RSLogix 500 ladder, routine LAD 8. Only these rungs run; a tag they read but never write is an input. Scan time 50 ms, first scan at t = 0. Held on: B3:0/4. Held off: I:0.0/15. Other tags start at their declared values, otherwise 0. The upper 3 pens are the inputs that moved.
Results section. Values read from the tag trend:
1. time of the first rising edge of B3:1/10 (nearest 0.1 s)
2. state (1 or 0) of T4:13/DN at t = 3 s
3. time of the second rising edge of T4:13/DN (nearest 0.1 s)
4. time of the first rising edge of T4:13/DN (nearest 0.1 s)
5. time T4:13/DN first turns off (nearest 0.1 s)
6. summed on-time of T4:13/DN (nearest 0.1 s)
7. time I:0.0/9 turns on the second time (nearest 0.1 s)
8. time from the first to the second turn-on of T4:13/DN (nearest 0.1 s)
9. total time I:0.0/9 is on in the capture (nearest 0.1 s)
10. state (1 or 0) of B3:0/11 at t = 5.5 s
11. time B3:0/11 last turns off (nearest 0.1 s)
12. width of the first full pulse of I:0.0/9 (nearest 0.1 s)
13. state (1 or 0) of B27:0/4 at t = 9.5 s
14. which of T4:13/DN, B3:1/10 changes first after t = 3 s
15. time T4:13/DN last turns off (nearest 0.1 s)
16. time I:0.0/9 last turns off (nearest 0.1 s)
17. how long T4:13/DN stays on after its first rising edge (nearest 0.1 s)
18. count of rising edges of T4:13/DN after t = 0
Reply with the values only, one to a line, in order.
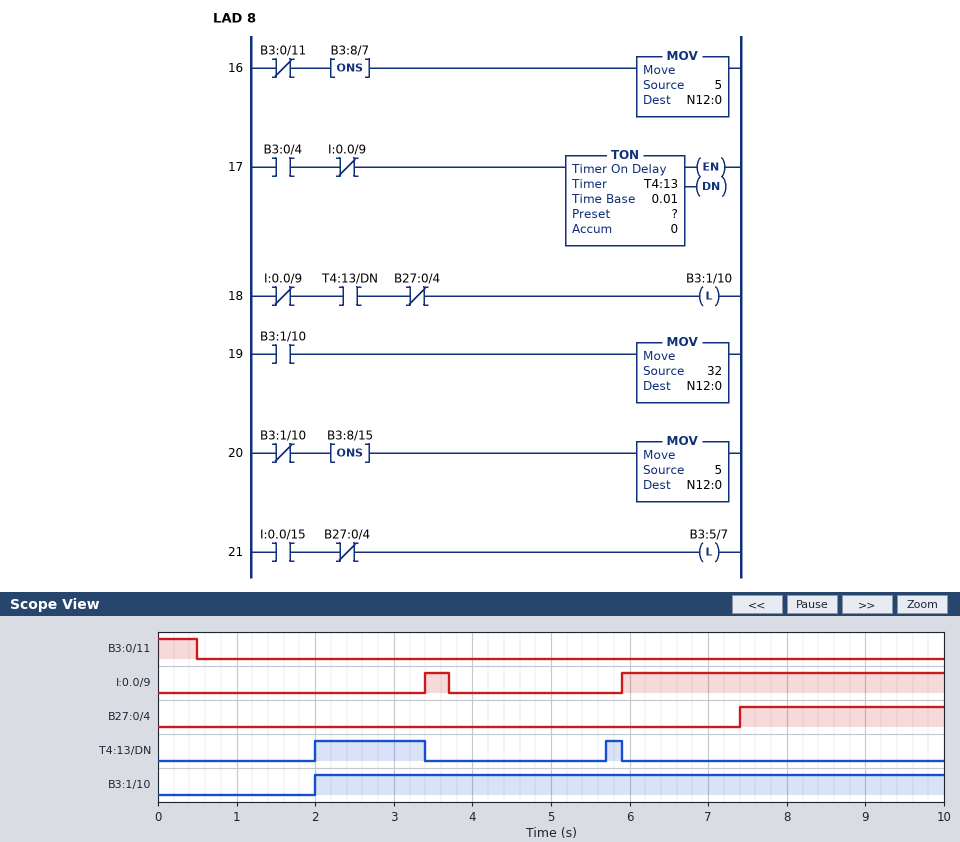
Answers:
2.0 s
1
5.7 s
2.0 s
3.4 s
1.6 s
5.9 s
3.7 s
4.4 s
0
0.5 s
0.3 s
1
T4:13/DN
5.9 s
3.7 s
1.4 s
2
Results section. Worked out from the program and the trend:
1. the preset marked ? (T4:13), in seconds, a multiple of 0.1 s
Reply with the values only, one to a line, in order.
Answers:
2.0 s
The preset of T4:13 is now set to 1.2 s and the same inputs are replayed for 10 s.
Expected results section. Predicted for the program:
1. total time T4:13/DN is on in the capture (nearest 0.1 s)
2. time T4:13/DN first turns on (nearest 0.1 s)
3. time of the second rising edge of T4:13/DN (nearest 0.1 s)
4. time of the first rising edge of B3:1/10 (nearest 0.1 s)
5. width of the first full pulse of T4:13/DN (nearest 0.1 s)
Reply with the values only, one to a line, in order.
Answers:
3.2 s
1.2 s
4.9 s
1.2 s
2.2 s
